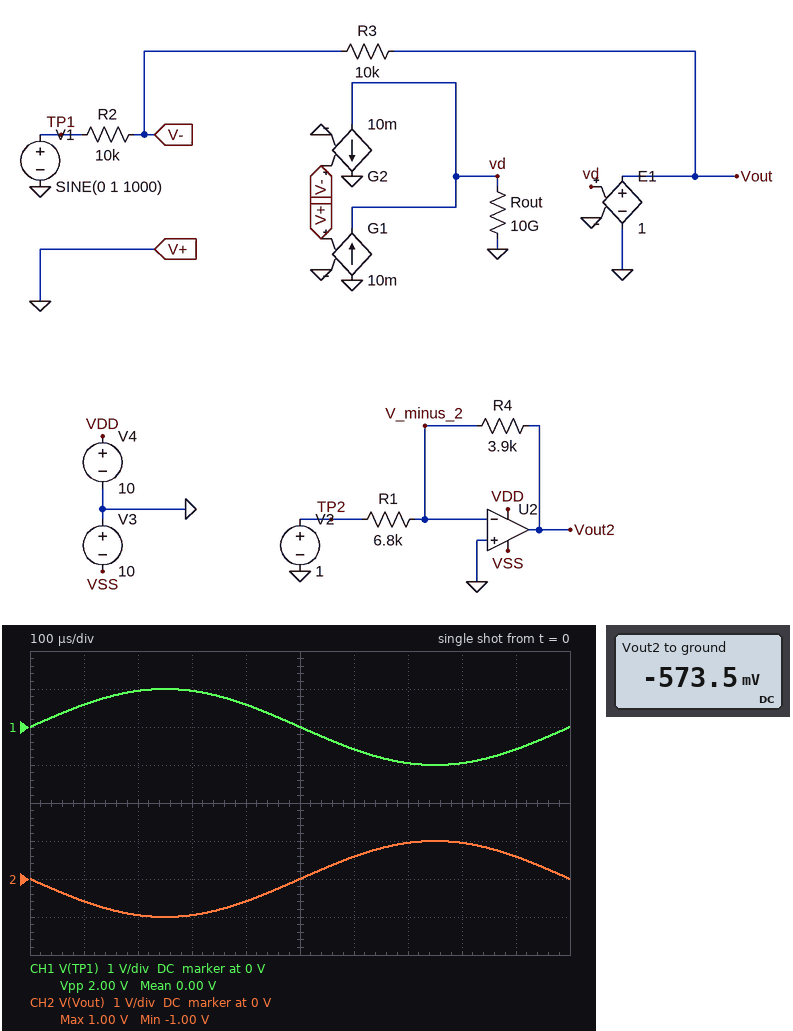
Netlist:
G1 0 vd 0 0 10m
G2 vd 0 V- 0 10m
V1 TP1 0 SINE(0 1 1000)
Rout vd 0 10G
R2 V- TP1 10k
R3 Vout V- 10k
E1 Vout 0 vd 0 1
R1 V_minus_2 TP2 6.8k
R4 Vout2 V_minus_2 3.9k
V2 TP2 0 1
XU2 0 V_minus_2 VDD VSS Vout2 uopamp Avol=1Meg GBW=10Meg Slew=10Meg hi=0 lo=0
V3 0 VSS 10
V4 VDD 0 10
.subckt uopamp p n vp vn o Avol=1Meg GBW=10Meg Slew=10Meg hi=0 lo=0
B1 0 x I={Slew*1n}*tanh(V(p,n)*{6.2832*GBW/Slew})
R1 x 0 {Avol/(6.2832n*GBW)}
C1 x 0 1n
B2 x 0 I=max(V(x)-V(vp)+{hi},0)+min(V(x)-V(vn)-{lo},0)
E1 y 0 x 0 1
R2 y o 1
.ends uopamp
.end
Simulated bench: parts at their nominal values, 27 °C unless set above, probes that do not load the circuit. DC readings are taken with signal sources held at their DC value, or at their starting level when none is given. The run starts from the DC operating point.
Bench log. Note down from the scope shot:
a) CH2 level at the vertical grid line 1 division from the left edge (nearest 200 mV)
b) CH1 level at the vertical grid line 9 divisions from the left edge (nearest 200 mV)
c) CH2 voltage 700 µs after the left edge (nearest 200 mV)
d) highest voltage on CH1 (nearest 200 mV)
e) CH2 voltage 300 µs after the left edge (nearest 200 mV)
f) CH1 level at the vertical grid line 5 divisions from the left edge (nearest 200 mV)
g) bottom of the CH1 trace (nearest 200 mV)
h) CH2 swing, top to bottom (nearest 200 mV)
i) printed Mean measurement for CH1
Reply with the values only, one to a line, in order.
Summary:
-600 mV
-600 mV
1.0 V
1.0 V
-1.0 V
0 V
-1.0 V
2.0 V
0.00 V
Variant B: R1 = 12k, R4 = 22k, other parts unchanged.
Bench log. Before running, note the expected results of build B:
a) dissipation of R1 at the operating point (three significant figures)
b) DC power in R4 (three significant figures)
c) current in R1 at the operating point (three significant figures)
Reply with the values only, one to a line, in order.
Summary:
83.3 µW
153 µW
83.3 µA
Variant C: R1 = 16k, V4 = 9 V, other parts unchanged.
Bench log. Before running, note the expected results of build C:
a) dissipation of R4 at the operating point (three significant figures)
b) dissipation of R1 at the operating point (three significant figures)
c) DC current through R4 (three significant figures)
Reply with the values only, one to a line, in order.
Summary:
15.2 µW
62.5 µW
62.5 µA
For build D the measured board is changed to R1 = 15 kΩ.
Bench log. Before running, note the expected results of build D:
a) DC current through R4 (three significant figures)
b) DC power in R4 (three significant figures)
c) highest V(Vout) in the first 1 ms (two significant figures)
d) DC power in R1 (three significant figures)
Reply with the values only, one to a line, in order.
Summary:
66.7 µA
17.3 µW
1.0 V
66.7 µW
